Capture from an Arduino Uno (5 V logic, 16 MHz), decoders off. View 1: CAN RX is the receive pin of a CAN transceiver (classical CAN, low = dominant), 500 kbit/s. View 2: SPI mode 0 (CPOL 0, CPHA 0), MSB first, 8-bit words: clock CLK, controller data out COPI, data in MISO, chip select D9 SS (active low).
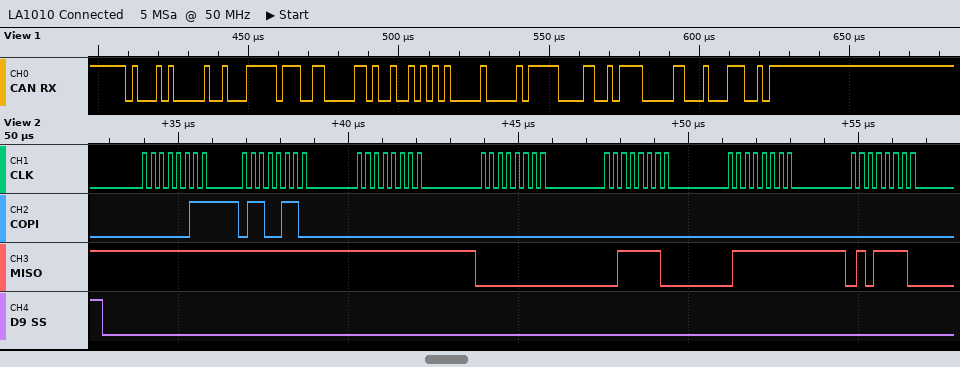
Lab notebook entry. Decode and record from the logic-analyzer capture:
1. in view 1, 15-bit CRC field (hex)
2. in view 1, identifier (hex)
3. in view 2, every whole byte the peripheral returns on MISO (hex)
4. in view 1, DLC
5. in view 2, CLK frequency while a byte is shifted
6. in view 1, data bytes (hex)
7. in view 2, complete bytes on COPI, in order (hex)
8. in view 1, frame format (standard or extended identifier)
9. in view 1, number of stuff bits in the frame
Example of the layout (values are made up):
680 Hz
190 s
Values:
0x111C
0x450
FF FF FF 00 3E 7F 5E
8
4 MHz
FF 30 52 55 00 1F 19 78
03 66 00 00 00 00 00
standard
7
